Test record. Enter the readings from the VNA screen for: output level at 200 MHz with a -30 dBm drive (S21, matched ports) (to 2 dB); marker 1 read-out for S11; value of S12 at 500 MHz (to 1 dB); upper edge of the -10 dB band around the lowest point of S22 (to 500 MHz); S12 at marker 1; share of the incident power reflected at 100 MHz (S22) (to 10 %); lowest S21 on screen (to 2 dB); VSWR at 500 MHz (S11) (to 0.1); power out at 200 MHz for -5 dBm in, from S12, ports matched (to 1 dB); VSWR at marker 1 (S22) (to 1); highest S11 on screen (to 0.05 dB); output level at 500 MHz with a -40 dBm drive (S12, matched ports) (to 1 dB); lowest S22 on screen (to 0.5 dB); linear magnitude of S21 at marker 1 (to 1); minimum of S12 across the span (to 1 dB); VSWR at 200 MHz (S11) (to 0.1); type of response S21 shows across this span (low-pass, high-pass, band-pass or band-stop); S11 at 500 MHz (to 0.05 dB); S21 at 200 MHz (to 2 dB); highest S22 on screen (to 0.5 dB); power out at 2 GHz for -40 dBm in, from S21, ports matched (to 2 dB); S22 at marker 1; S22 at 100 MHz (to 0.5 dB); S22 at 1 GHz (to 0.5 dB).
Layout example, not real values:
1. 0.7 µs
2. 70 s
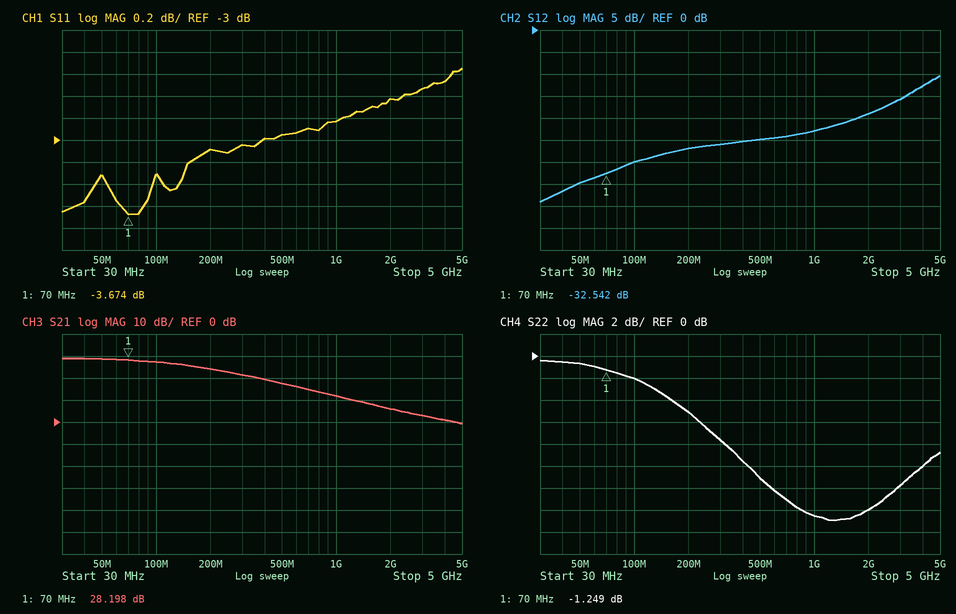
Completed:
1. -6 dBm
2. -3.674 dB
3. -25 dB
4. 4.0 GHz
5. -32.542 dB
6. 60 %
7. 0 dB
8. 5.9
9. -32 dBm
10. 14
11. -2.35 dB
12. -65 dBm
13. -15.0 dB
14. 26
15. -39 dB
16. 5.7
17. low-pass
18. -2.95 dB
19. 24 dB
20. -0.5 dB
21. -34 dBm
22. -1.249 dB
23. -2.0 dB
24. -14.5 dB
